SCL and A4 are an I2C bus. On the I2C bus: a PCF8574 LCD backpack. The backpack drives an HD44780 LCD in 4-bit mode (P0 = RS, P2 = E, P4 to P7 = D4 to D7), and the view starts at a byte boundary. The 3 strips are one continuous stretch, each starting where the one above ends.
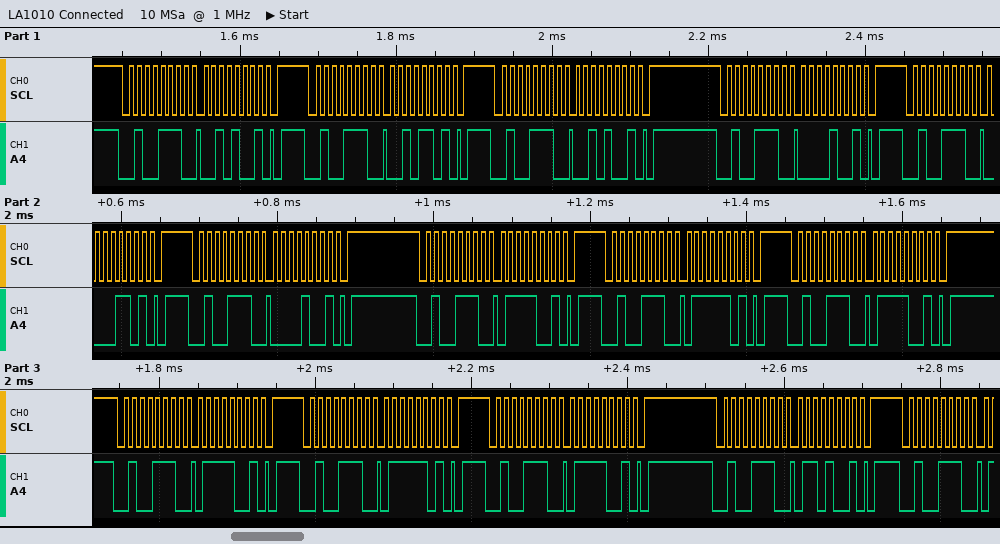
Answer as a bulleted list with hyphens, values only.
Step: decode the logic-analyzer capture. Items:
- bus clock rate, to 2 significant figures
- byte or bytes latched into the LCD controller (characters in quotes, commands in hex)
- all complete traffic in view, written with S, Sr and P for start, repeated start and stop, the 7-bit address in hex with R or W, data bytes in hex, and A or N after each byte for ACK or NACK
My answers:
- 100 kHz
- ' ' 'w'
- S 27W A 29 A P S 27W A 2D A P S 27W A 29 A P S 27W A 09 A P S 27W A 0D A P S 27W A 09 A P S 27W A 79 A P S 27W A 7D A P S 27W A 79 A P S 27W A 79 A P S 27W A 7D A P S 27W A 79 A P S 27W A 69 A P S 27W A
